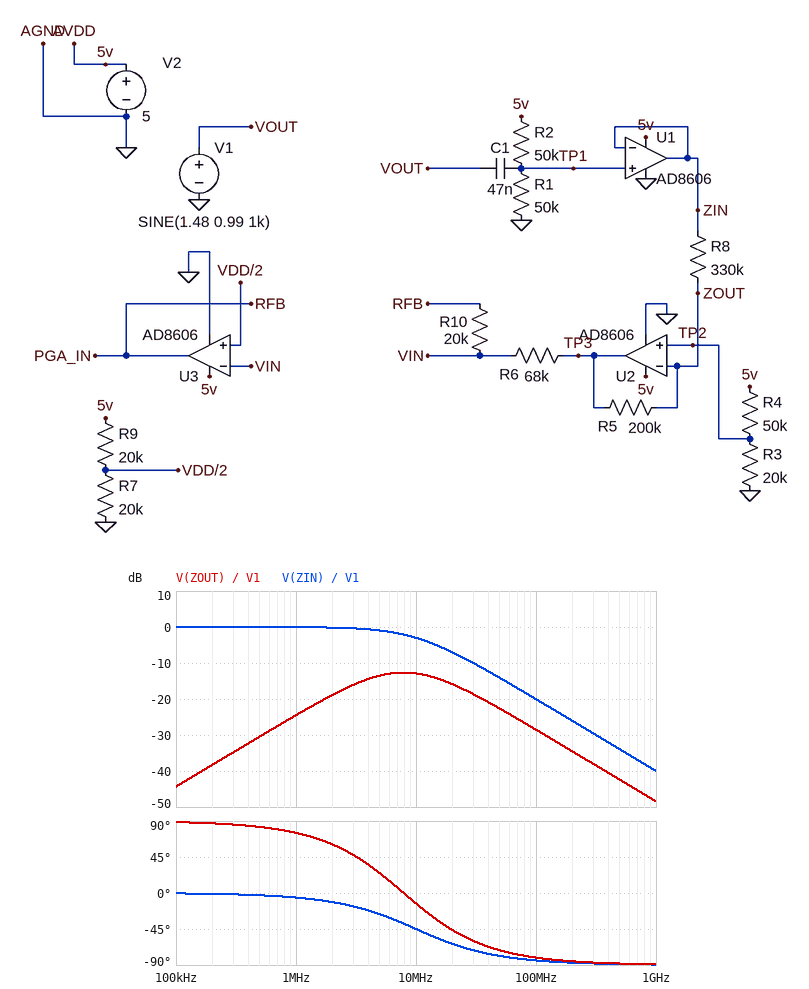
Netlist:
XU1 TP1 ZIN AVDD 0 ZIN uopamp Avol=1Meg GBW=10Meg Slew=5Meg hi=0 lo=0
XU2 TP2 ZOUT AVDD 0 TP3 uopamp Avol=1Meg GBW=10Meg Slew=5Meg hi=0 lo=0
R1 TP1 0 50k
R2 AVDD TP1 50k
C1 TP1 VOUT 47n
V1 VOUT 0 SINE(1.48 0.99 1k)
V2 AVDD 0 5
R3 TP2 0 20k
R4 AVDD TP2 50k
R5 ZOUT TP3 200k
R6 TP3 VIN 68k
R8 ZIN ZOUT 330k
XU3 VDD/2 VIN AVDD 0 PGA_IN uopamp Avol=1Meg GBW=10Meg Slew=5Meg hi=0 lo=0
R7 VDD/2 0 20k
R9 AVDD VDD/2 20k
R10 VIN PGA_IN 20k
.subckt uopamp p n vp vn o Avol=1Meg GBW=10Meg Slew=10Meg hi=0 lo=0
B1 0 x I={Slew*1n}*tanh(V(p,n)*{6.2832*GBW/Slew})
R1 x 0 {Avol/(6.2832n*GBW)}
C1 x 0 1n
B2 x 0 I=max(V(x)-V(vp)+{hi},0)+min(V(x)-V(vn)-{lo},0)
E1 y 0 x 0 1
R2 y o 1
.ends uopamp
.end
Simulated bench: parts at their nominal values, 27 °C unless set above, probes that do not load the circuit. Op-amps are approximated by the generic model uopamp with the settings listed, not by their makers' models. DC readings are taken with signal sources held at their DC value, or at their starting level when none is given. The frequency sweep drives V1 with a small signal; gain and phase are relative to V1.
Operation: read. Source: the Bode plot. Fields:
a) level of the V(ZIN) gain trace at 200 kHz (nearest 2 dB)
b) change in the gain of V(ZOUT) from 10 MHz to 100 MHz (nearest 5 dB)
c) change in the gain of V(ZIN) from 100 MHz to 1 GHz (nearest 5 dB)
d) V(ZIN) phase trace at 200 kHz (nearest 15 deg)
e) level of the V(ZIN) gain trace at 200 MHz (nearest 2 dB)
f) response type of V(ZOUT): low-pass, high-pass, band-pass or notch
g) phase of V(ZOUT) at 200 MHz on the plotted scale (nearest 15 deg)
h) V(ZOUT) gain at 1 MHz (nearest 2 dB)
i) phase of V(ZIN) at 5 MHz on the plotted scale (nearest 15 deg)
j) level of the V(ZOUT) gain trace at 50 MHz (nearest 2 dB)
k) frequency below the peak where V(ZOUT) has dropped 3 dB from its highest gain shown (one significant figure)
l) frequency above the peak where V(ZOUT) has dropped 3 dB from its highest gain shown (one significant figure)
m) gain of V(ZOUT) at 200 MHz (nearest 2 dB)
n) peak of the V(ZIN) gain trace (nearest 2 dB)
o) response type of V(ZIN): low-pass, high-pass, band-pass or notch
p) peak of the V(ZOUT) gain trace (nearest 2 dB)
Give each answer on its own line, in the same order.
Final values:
0 dB
-15 dB
-20 dB
0 deg
-26 dB
band-pass
-90 deg
-24 dB
-30 deg
-22 dB
3 MHz
20 MHz
-34 dB
0 dB
low-pass
-12 dB
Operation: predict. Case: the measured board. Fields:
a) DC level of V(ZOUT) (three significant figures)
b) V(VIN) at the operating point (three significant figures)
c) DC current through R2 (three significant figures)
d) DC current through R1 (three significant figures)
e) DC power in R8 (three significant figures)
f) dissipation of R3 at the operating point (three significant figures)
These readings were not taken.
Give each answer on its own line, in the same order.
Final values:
1.43 V
2.50 V
50.0 µA
50.0 µA
3.48 µW
102 µW
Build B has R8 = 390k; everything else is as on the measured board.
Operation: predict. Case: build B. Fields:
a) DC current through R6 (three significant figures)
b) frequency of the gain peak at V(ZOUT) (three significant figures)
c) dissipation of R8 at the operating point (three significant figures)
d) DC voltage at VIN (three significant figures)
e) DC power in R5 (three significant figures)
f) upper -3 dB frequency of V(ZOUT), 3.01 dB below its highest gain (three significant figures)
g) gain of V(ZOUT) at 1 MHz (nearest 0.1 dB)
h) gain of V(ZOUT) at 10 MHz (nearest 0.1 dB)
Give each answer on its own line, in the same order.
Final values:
23.8 µA
8.13 MHz
2.94 µW
2.50 V
1.51 µW
19.9 MHz
-25.9 dB
-14.0 dB
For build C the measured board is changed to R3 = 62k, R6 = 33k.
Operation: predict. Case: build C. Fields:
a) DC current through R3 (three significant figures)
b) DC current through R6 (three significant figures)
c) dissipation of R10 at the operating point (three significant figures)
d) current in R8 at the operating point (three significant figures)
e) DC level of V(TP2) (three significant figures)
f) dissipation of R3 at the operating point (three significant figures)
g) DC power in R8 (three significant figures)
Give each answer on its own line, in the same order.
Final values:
44.6 µA
13.0 µA
3.40 µW
812 nA
2.77 V
124 µW
217 nW
